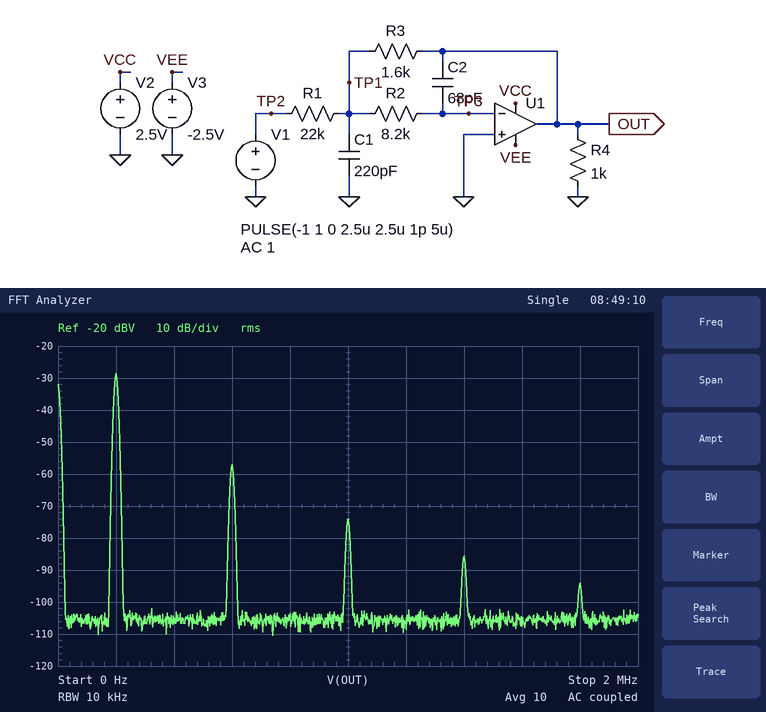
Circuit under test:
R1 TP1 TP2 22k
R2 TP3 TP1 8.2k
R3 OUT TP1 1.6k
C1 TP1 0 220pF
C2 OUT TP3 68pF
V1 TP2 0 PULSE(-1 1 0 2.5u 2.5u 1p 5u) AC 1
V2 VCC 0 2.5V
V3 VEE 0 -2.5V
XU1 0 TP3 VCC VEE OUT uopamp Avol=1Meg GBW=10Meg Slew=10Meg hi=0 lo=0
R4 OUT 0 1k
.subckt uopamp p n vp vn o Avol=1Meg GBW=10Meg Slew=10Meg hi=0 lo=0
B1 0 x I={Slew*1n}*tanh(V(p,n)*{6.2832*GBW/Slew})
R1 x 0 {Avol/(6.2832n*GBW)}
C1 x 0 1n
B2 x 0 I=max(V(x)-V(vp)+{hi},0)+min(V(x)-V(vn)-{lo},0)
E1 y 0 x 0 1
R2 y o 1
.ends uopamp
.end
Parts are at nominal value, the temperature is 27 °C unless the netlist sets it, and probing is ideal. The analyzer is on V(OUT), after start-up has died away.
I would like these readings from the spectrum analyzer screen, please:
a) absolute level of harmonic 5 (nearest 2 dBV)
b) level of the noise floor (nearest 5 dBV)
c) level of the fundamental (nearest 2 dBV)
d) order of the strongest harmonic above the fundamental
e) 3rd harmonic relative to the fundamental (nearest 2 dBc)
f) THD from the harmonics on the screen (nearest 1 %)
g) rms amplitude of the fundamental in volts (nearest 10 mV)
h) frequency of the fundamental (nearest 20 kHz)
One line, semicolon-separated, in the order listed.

-74 dBV; -105 dBV; -28 dBV; 3; -28 dBc; 4 %; 40 mV; 200 kHz
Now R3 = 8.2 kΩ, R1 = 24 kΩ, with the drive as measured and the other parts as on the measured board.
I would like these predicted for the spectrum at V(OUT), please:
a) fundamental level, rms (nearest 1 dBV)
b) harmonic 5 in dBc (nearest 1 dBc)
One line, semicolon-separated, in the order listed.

-19 dBV; -55 dBc
